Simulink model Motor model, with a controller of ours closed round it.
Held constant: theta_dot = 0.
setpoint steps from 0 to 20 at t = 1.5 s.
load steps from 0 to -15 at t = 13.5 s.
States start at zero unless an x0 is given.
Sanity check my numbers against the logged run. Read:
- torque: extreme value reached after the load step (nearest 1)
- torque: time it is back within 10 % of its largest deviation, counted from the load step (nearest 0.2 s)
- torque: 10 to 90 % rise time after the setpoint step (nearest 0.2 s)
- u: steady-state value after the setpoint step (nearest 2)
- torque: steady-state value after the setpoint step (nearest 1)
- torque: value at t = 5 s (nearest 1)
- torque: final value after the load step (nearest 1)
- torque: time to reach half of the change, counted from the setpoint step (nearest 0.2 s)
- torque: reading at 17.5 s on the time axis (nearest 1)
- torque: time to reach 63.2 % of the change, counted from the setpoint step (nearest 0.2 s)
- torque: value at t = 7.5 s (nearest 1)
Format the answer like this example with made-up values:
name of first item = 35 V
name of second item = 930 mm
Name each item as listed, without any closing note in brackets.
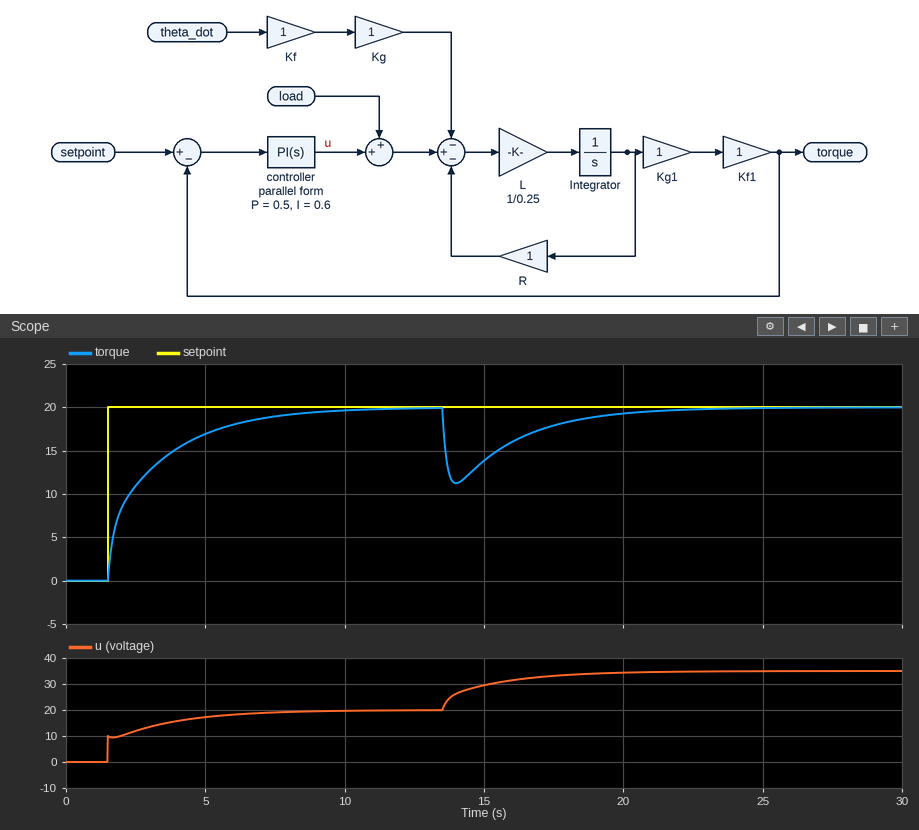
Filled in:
torque: extreme value reached after the load step = 11
torque: time it is back within 10 % of its largest deviation, counted from the load step = 6.0 s
torque: 10 to 90 % rise time after the setpoint step = 4.4 s
u: steady-state value after the setpoint step = 20
torque: steady-state value after the setpoint step = 20
torque: value at t = 5 s = 17
torque: final value after the load step = 20
torque: time to reach half of the change, counted from the setpoint step = 0.8 s
torque: reading at 17.5 s on the time axis = 18
torque: time to reach 63.2 % of the change, counted from the setpoint step = 1.4 s
torque: value at t = 7.5 s = 19
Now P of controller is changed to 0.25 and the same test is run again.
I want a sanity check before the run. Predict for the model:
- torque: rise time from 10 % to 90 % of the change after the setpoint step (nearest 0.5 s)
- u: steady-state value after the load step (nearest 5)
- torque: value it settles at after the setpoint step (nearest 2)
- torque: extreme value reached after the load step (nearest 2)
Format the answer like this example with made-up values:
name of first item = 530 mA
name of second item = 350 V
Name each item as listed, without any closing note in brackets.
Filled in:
torque: rise time from 10 % to 90 % of the change after the setpoint step = 4.0 s
u: steady-state value after the load step = 35
torque: value it settles at after the setpoint step = 20
torque: extreme value reached after the load step = 10
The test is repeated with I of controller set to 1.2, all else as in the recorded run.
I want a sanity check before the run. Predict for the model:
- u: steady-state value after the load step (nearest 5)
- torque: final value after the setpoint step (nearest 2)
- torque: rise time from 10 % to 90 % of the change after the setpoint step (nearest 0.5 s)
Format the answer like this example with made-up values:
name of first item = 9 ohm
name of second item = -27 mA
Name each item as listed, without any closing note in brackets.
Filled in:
u: steady-state value after the load step = 35
torque: final value after the setpoint step = 20
torque: rise time from 10 % to 90 % of the change after the setpoint step = 2.0 s
